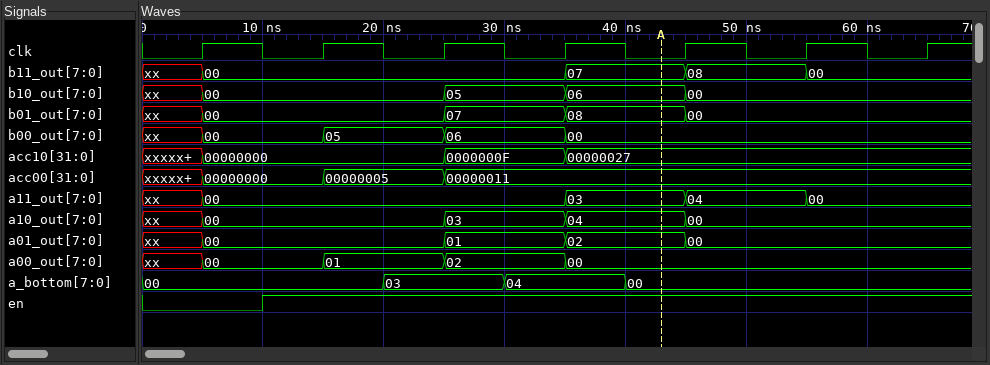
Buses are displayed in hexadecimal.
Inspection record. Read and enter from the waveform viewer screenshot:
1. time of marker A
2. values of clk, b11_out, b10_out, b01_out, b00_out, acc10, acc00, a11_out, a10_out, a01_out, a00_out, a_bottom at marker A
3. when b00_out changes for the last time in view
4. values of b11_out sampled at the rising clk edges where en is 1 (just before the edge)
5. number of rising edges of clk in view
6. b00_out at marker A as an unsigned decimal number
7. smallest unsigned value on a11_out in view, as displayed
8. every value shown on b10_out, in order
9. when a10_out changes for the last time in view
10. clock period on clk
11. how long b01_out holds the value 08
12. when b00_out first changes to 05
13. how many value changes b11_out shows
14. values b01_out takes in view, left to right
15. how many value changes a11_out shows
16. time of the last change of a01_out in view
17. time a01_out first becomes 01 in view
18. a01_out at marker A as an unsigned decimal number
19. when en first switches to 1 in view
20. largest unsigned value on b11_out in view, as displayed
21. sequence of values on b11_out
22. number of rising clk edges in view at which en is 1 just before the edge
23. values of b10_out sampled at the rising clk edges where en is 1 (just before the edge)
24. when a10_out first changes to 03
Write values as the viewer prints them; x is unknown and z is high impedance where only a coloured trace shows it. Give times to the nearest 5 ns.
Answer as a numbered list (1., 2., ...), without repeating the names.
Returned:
1. 45 ns
2. clk=0, b11_out=07, b10_out=06, b01_out=08, b00_out=00, acc10=00000027, acc00=00000011, a11_out=03, a10_out=04, a01_out=02, a00_out=00, a_bottom=00
3. 35 ns
4. 00, 00, 00, 07, 08, 00
5. 7
6. 0
7. 00
8. xx, 00, 05, 06, 00
9. 45 ns
10. 10 ns
11. 10 ns
12. 15 ns
13. 4
14. xx, 00, 07, 08, 00
15. 4
16. 45 ns
17. 25 ns
18. 2
19. 10 ns
20. 08
21. xx, 00, 07, 08, 00
22. 6
23. 00, 00, 05, 06, 00, 00
24. 25 ns
